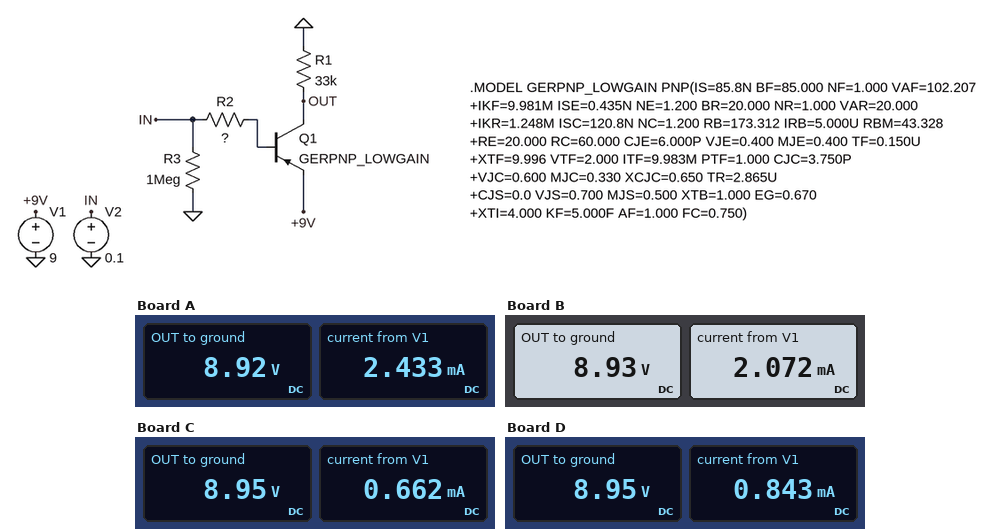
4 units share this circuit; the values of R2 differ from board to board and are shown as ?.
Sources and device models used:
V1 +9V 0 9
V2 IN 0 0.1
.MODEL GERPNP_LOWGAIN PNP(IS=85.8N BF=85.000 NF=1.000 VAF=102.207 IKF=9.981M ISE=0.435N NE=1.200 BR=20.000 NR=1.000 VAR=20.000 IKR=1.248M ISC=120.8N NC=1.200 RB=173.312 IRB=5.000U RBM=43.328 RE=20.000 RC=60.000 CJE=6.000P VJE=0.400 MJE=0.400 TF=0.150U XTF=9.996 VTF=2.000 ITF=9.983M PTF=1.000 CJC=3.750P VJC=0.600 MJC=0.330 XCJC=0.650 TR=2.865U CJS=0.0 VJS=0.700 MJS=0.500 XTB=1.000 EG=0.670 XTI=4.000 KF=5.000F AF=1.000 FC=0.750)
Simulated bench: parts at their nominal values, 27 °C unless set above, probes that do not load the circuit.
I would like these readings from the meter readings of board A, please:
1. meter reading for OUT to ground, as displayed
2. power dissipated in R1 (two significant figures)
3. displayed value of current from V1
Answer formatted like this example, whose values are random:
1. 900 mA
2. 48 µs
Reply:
1. 8.92 V
2. 2.4 mW
3. 2.433 mA
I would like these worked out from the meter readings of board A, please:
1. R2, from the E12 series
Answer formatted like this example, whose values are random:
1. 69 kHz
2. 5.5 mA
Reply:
1. 3.9 kΩ
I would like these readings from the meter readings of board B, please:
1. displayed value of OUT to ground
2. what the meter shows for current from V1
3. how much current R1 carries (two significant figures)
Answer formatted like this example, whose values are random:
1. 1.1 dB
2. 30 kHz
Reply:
1. 8.93 V
2. 2.072 mA
3. 270 µA
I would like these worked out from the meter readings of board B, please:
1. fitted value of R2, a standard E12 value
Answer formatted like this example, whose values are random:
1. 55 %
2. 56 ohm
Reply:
1. 4.7 kΩ
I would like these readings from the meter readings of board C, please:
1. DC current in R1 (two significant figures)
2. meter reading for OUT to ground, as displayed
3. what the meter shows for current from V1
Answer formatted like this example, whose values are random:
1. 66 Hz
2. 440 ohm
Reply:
1. 270 µA
2. 8.95 V
3. 0.662 mA
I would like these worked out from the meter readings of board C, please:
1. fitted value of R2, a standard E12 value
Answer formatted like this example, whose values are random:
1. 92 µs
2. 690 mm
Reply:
1. 22 kΩ
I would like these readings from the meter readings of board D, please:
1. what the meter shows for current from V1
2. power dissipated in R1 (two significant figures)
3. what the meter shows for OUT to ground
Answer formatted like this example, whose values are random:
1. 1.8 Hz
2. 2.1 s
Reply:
1. 0.843 mA
2. 2.4 mW
3. 8.95 V
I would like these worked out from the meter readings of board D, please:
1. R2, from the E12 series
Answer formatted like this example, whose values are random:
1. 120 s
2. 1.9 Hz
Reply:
1. 15 kΩ
